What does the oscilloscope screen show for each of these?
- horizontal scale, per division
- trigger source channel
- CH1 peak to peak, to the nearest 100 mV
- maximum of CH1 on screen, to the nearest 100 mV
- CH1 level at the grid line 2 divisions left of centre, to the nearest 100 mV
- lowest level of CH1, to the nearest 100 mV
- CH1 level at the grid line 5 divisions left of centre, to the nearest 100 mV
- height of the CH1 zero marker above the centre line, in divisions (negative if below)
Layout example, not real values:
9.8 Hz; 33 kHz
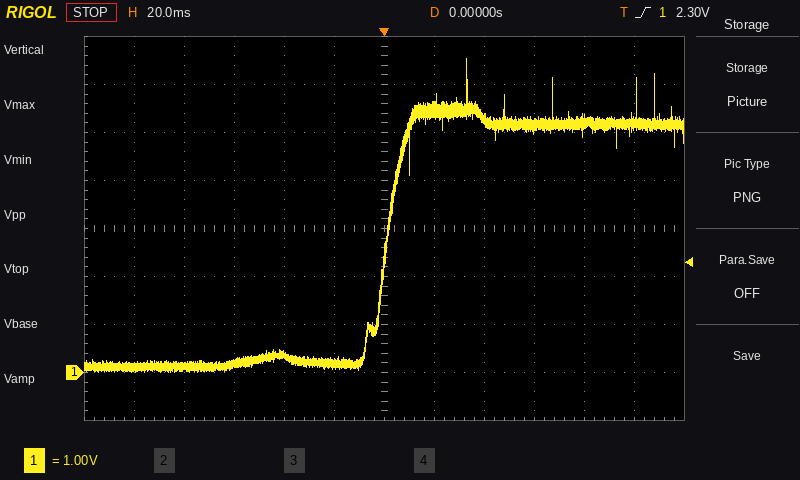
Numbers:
20 ms; CH1; 6.5 V; 6.5 V; 400 mV; 0.0 V; 100 mV; -3.0 div
